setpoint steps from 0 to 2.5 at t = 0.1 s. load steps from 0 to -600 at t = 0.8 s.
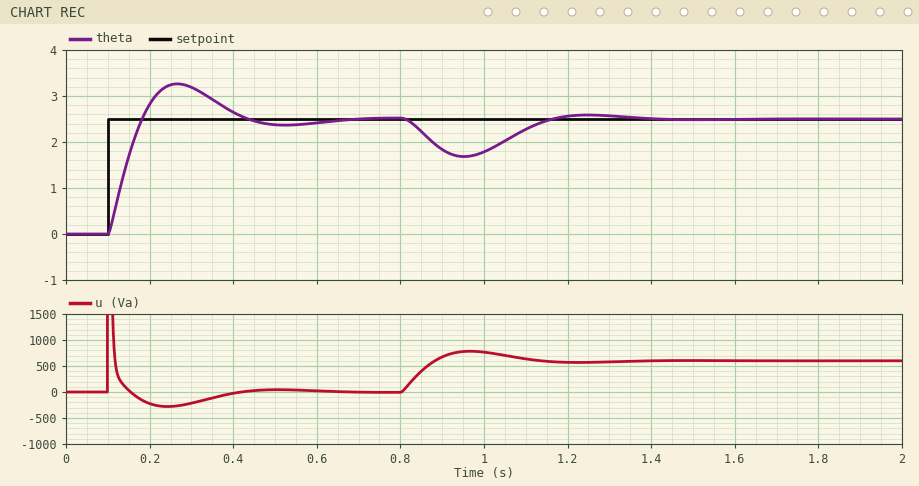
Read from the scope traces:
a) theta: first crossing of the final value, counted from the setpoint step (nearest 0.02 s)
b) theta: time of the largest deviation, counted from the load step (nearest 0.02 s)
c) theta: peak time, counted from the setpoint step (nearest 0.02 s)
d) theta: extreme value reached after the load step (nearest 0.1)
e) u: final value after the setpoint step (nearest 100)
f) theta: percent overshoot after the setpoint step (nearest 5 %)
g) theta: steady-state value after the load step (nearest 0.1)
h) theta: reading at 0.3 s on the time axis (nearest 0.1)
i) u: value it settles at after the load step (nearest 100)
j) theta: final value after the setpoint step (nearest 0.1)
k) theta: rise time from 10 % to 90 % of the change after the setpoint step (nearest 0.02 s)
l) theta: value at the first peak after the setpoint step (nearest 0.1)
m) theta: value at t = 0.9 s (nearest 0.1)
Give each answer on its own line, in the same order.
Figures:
0.08 s
0.16 s
0.16 s
1.7
0
30 %
2.5
3.2
600
2.5
0.06 s
3.3
1.8
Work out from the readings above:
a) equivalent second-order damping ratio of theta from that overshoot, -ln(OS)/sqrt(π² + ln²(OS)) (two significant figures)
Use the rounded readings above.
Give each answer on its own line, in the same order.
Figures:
0.36
